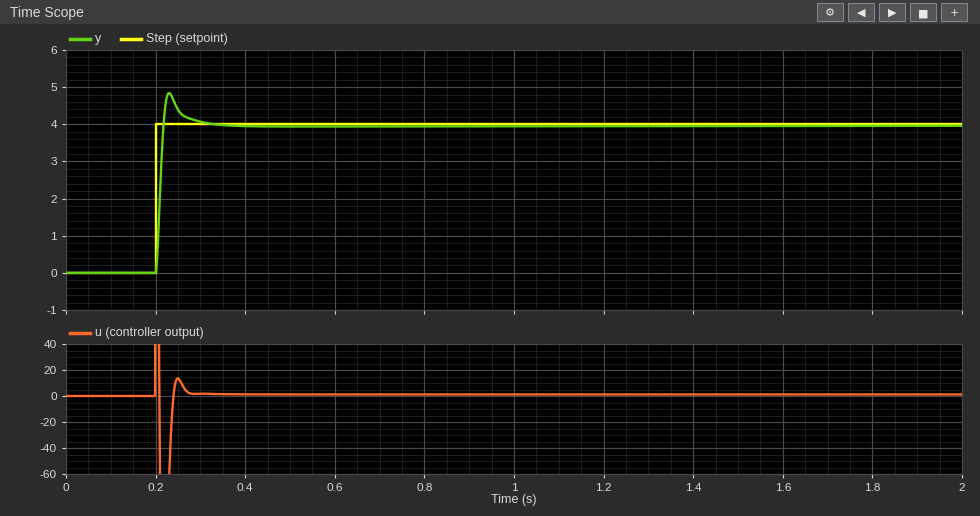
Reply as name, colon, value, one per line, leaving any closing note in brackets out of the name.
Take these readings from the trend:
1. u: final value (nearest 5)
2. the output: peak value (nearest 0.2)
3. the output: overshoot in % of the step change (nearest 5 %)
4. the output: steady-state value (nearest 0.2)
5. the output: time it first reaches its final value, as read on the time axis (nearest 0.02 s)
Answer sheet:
u: final value: 0
the output: peak value: 4.8
the output: overshoot in % of the step change: 20 %
the output: steady-state value: 4.0
the output: time it first reaches its final value, as read on the time axis: 0.22 s
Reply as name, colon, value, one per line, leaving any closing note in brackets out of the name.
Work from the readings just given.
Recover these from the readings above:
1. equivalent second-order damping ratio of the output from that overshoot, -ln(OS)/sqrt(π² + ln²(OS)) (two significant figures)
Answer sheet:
equivalent second-order damping ratio of the output from that overshoot, -ln(OS)/sqrt(π² + ln²(OS)): 0.46
